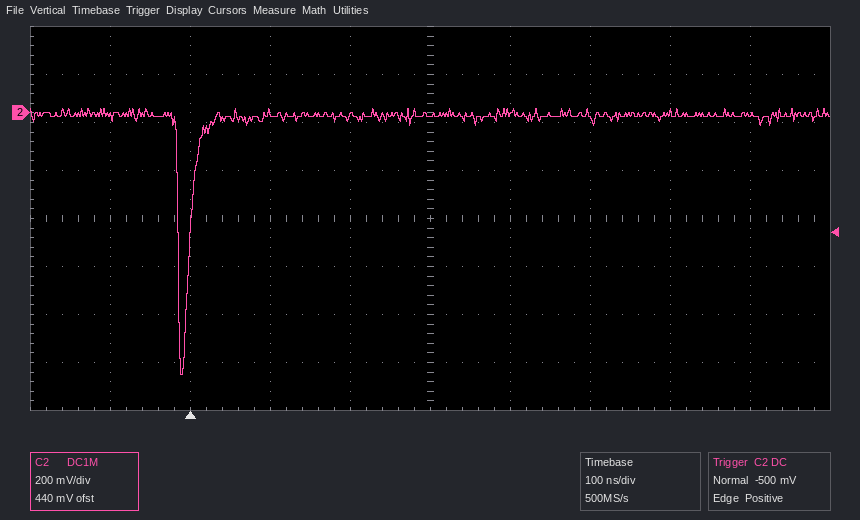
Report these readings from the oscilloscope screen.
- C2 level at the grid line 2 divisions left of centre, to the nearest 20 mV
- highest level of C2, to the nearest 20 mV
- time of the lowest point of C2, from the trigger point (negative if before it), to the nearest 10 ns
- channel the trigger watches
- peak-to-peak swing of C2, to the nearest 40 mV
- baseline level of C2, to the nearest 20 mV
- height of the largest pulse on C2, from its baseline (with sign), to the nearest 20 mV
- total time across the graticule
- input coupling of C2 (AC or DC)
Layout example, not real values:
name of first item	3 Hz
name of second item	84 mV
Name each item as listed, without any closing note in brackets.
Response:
C2 level at the grid line 2 divisions left of centre, to the nearest 20 mV	0 mV
highest level of C2, to the nearest 20 mV	20 mV
time of the lowest point of C2, from the trigger point (negative if before it), to the nearest 10 ns	-10 ns
channel the trigger watches	C2
peak-to-peak swing of C2, to the nearest 40 mV	1.12 V
baseline level of C2, to the nearest 20 mV	-20 mV
height of the largest pulse on C2, from its baseline (with sign), to the nearest 20 mV	-1.08 V
total time across the graticule	1 µs
input coupling of C2	DC
